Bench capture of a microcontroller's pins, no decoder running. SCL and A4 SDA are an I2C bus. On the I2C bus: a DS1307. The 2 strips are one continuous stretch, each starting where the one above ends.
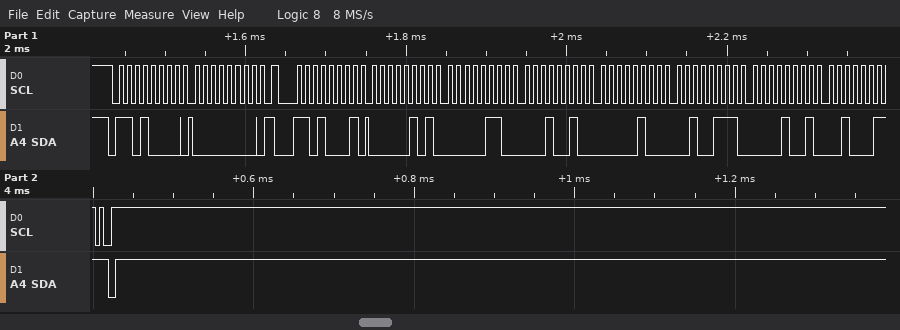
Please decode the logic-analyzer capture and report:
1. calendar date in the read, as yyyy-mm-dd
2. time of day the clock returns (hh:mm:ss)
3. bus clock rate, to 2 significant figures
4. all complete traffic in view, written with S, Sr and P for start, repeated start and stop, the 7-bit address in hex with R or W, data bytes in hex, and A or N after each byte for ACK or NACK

2023-09-27
12:06:05
100 kHz
S 68W A 00 A Sr 68R A 05 A 06 A 12 A 04 A 27 A 09 A 23 N P
